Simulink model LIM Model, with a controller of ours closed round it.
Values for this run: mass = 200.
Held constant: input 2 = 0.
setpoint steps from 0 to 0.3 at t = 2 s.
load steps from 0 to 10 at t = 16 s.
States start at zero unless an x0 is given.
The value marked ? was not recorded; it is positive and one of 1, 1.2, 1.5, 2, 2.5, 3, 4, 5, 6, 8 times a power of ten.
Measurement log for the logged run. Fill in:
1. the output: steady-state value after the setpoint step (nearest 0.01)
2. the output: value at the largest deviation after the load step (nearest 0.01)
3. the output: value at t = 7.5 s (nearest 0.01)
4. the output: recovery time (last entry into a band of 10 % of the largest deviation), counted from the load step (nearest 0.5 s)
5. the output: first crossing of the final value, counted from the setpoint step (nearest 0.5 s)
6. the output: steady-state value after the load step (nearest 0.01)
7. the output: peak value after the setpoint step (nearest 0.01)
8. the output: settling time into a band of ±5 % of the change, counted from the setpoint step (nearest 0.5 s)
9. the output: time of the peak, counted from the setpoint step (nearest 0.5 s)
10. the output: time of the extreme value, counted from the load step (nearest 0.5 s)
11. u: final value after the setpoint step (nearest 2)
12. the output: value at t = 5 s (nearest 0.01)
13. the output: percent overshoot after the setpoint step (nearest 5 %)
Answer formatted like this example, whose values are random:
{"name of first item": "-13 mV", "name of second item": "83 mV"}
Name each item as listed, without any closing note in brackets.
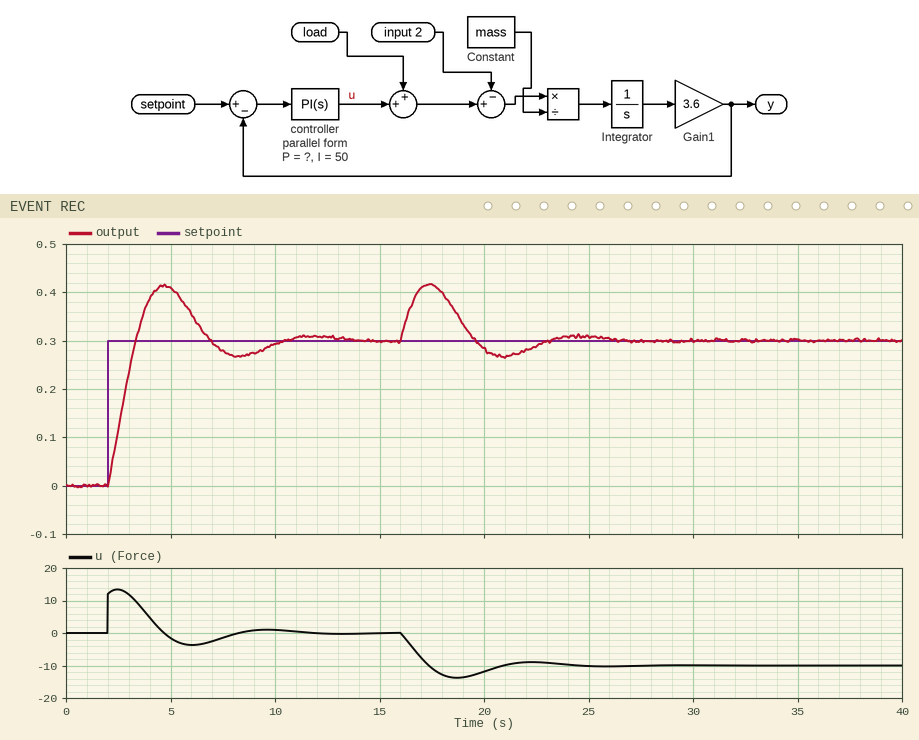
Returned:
{"the output: steady-state value after the setpoint step": "0.30", "the output: value at the largest deviation after the load step": "0.42", "the output: value at t = 7.5 s": "0.28", "the output: recovery time (last entry into a band of 10 % of the largest deviation), counted from the load step": "6.5 s", "the output: first crossing of the final value, counted from the setpoint step": "1.5 s", "the output: steady-state value after the load step": "0.30", "the output: peak value after the setpoint step": "0.41", "the output: settling time into a band of ±5 % of the change, counted from the setpoint step": "7.5 s", "the output: time of the peak, counted from the setpoint step": "2.5 s", "the output: time of the extreme value, counted from the load step": "1.5 s", "u: final value after the setpoint step": "0", "the output: value at t = 5 s": "0.41", "the output: percent overshoot after the setpoint step": "40 %"}
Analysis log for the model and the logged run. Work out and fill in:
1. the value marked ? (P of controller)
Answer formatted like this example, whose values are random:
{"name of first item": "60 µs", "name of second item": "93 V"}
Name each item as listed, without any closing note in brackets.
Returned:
{"the value marked ?": "40"}
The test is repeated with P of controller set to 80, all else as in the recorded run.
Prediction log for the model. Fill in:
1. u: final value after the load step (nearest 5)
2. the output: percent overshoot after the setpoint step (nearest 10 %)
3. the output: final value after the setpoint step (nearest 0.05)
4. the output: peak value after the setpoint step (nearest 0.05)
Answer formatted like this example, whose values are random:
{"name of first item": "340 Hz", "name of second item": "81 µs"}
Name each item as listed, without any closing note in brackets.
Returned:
{"u: final value after the load step": "-10", "the output: percent overshoot after the setpoint step": "20 %", "the output: final value after the setpoint step": "0.30", "the output: peak value after the setpoint step": "0.35"}
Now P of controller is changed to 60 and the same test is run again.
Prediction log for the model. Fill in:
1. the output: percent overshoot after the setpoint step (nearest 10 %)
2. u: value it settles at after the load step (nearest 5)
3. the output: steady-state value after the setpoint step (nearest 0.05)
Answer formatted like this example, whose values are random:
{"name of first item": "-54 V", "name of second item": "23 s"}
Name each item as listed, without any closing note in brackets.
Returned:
{"the output: percent overshoot after the setpoint step": "30 %", "u: value it settles at after the load step": "-10", "the output: steady-state value after the setpoint step": "0.30"}
